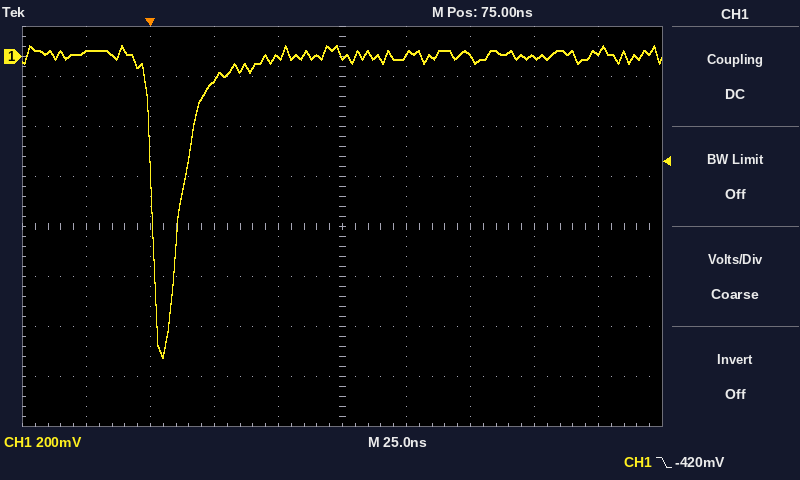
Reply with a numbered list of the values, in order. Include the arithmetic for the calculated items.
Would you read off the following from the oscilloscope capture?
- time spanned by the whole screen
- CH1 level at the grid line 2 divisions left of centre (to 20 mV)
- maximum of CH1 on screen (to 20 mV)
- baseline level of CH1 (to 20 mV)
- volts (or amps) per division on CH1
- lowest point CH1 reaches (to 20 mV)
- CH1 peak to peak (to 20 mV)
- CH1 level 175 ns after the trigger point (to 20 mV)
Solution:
1. 250 ns
2. -100 mV
3. 40 mV
4. 0 mV
5. 200 mV
6. -1.20 V
7. 40 mV − (-1.20 V) = 1.24 V
8. 20 mV
